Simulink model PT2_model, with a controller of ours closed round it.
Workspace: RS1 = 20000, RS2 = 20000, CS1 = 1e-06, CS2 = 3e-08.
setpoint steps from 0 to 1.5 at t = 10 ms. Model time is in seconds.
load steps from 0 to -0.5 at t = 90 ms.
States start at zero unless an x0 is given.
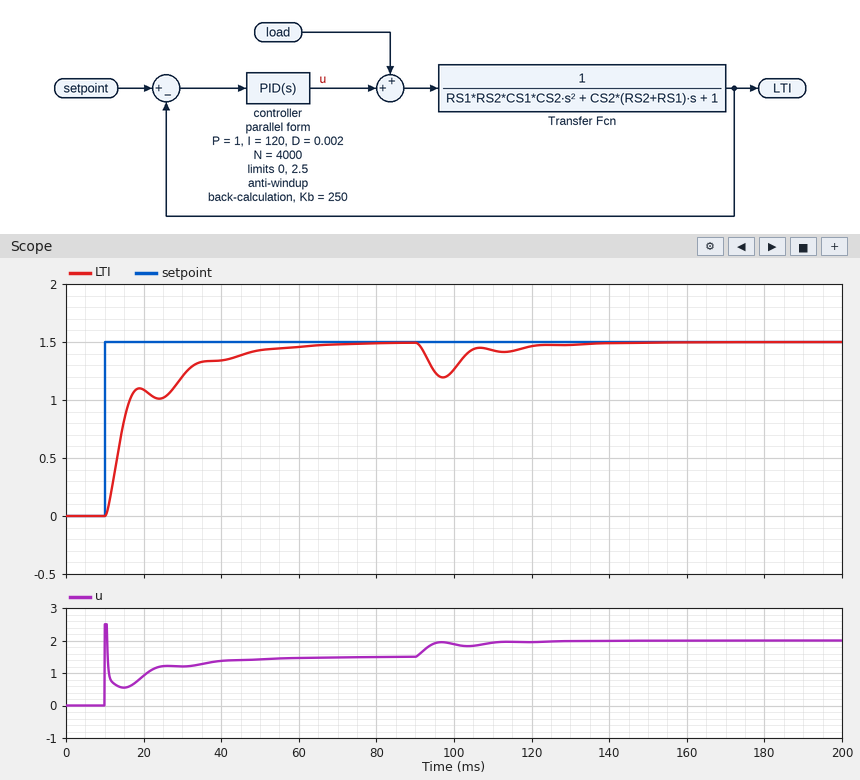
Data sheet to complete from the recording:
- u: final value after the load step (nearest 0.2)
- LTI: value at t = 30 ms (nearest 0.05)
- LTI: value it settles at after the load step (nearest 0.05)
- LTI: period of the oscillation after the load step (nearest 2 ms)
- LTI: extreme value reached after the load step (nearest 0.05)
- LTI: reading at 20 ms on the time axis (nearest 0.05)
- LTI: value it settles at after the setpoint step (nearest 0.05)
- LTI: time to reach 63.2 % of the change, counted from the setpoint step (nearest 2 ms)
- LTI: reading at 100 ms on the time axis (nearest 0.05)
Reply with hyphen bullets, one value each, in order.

- 2.0
- 1.20
- 1.50
- 16 ms
- 1.20
- 1.10
- 1.50
- 6 ms
- 1.25
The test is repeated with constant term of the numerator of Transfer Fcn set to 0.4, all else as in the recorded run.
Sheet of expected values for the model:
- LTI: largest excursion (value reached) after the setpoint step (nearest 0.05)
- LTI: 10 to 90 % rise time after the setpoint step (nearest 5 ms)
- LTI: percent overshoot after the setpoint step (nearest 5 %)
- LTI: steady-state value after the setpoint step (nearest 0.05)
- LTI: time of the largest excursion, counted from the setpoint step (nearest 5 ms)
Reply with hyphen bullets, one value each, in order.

- 1.10
- 20 ms
- 10 %
- 1.00
- 30 ms
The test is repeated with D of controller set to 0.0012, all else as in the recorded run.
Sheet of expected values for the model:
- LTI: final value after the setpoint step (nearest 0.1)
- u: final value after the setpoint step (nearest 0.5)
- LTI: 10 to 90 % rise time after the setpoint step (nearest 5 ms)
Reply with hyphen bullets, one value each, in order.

- 1.5
- 1.5
- 20 ms
